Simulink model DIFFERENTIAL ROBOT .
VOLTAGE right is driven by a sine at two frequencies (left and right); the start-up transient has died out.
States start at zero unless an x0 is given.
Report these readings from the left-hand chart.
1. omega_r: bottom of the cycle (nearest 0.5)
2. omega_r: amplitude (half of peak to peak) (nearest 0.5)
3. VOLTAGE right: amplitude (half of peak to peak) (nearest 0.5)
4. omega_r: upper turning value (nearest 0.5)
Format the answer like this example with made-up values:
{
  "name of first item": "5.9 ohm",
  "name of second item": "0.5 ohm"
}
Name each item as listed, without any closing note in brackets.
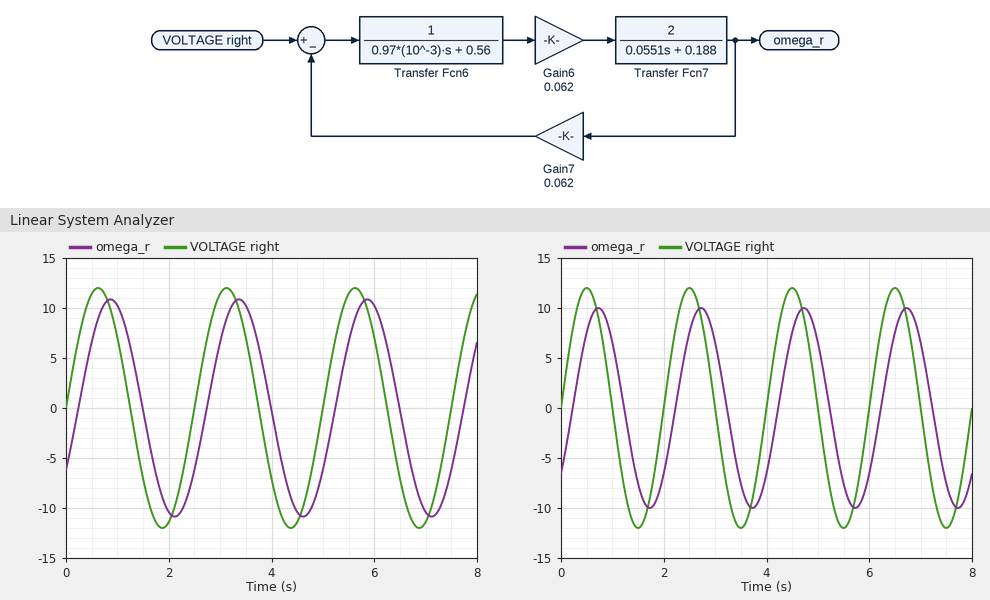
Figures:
{
  "omega_r: bottom of the cycle": "-11.0",
  "omega_r: amplitude (half of peak to peak)": "11.0",
  "VOLTAGE right: amplitude (half of peak to peak)": "12.0",
  "omega_r: upper turning value": "11.0"
}
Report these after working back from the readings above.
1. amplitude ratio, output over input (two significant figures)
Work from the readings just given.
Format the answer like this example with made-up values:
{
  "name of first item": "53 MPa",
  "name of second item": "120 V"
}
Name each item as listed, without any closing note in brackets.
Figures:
{
  "amplitude ratio, output over input": "0.92"
}
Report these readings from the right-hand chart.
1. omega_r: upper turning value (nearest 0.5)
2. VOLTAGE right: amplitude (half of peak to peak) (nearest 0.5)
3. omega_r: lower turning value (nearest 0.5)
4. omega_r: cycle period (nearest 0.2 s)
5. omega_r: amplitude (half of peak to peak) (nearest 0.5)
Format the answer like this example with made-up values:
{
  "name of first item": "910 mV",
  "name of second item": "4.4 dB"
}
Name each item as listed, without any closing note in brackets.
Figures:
{
  "omega_r: upper turning value": "10.0",
  "VOLTAGE right: amplitude (half of peak to peak)": "12.0",
  "omega_r: lower turning value": "-10.0",
  "omega_r: cycle period": "2.0 s",
  "omega_r: amplitude (half of peak to peak)": "10.0"
}
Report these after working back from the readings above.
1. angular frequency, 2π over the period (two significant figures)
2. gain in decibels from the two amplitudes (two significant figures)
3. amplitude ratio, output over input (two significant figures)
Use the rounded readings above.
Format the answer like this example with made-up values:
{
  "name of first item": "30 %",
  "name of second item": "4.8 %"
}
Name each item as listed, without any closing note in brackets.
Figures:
{
  "angular frequency, 2π over the period": "3.1 rad/s",
  "gain in decibels from the two amplitudes": "-1.6 dB",
  "amplitude ratio, output over input": "0.83"
}
